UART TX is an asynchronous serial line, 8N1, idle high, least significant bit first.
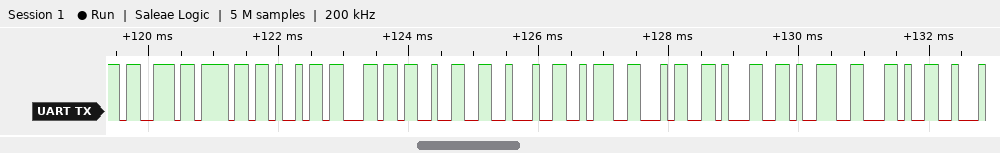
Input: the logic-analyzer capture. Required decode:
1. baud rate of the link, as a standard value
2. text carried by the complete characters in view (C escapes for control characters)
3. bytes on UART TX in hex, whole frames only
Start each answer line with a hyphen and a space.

- 9600 baud
- "soil2\":419,"
- 0x73 0x6F 0x69 0x6C 0x32 0x22 0x3A 0x34 0x31 0x39 0x2C
